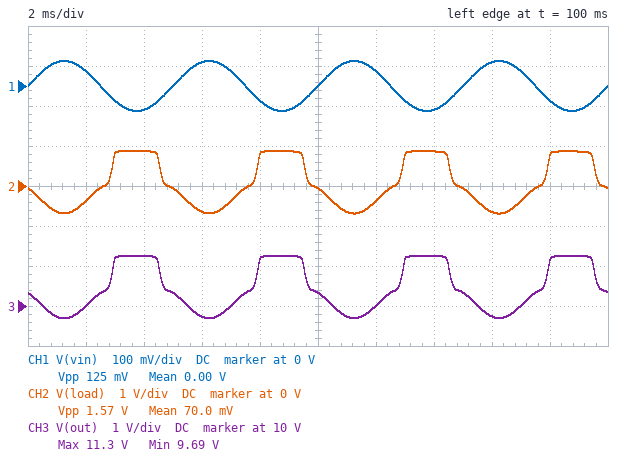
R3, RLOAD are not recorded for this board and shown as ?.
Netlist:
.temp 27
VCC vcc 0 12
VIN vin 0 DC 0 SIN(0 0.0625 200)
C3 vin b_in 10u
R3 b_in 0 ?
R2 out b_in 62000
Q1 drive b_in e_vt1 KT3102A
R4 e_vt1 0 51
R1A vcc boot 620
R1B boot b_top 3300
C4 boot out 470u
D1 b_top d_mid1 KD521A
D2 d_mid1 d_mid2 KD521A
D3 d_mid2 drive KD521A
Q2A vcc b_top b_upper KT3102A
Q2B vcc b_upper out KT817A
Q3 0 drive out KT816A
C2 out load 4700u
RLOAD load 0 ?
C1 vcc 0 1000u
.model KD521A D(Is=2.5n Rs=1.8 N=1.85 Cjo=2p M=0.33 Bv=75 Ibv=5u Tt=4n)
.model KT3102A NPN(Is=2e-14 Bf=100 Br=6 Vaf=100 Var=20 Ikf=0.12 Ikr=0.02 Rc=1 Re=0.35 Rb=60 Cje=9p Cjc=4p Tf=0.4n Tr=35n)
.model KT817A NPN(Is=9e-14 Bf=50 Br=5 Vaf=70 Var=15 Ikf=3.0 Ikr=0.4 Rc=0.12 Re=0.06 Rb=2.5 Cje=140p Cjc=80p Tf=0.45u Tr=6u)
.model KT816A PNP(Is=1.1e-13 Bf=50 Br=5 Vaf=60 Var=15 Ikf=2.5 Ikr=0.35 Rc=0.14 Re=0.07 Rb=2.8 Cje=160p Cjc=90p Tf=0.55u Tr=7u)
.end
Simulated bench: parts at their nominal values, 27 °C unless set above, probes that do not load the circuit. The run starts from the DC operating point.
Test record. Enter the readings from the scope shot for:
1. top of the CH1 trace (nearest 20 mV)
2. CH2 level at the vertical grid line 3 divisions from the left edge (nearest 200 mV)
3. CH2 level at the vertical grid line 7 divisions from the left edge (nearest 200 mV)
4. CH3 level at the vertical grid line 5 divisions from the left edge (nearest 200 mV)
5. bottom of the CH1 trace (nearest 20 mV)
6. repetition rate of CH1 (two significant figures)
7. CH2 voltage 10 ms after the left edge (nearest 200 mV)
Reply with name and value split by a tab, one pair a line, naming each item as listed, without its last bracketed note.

top of the CH1 trace	60 mV
CH2 level at the vertical grid line 3 divisions from the left edge	-600 mV
CH2 level at the vertical grid line 7 divisions from the left edge	800 mV
CH3 level at the vertical grid line 5 divisions from the left edge	10.4 V
bottom of the CH1 trace	-60 mV
repetition rate of CH1	200 Hz
CH2 voltage 10 ms after the left edge	0 V
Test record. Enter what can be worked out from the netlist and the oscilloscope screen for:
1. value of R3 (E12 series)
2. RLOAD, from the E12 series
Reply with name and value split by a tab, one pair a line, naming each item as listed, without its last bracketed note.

value of R3	3.9 kΩ
RLOAD, from the E12 series	22 Ω
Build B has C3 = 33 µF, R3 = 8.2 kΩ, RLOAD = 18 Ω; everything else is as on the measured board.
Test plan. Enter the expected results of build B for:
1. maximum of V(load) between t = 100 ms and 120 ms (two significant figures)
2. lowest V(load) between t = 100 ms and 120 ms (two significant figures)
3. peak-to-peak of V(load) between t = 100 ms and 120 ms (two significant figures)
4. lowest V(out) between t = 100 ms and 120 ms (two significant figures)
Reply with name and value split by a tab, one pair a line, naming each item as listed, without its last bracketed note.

maximum of V(load) between t = 100 ms and 120 ms	3.8 V
lowest V(load) between t = 100 ms and 120 ms	-1.4 V
peak-to-peak of V(load) between t = 100 ms and 120 ms	5.2 V
lowest V(out) between t = 100 ms and 120 ms	6.0 V
